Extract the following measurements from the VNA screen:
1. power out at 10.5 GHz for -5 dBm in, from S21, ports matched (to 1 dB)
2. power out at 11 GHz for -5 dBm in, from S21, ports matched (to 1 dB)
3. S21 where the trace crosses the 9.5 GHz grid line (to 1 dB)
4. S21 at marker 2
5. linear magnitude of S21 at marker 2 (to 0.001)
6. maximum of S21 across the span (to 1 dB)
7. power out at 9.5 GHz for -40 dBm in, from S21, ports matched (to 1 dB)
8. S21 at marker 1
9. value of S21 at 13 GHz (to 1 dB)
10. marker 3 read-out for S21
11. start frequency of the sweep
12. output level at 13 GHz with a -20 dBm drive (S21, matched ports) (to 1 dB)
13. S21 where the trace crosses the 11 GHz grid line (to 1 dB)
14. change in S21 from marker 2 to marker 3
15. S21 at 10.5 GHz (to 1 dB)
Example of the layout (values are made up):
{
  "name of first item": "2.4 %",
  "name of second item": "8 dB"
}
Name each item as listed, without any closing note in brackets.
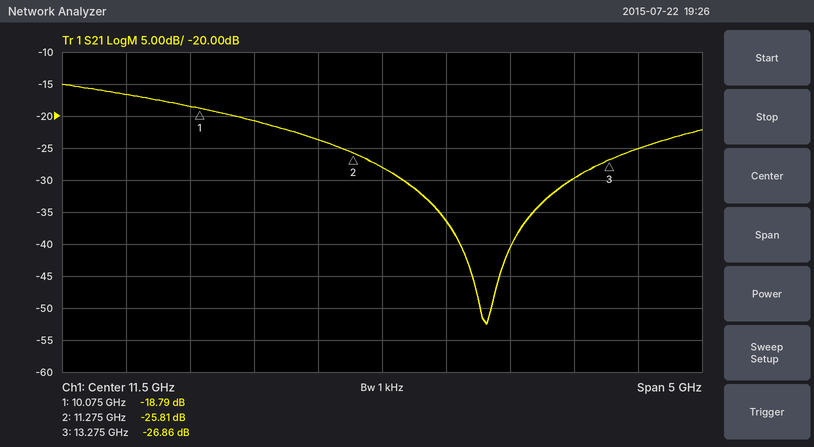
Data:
{
  "power out at 10.5 GHz for -5 dBm in, from S21, ports matched": "-26 dBm",
  "power out at 11 GHz for -5 dBm in, from S21, ports matched": "-29 dBm",
  "S21 where the trace crosses the 9.5 GHz grid line": "-17 dB",
  "S21 at marker 2": "-25.81 dB",
  "linear magnitude of S21 at marker 2": "0.051",
  "maximum of S21 across the span": "-15 dB",
  "power out at 9.5 GHz for -40 dBm in, from S21, ports matched": "-57 dBm",
  "S21 at marker 1": "-18.79 dB",
  "value of S21 at 13 GHz": "-30 dB",
  "marker 3 read-out for S21": "-26.86 dB",
  "start frequency of the sweep": "9 GHz",
  "output level at 13 GHz with a -20 dBm drive (S21, matched ports)": "-50 dBm",
  "S21 where the trace crosses the 11 GHz grid line": "-24 dB",
  "change in S21 from marker 2 to marker 3": "-1.05 dB",
  "S21 at 10.5 GHz": "-21 dB"
}
